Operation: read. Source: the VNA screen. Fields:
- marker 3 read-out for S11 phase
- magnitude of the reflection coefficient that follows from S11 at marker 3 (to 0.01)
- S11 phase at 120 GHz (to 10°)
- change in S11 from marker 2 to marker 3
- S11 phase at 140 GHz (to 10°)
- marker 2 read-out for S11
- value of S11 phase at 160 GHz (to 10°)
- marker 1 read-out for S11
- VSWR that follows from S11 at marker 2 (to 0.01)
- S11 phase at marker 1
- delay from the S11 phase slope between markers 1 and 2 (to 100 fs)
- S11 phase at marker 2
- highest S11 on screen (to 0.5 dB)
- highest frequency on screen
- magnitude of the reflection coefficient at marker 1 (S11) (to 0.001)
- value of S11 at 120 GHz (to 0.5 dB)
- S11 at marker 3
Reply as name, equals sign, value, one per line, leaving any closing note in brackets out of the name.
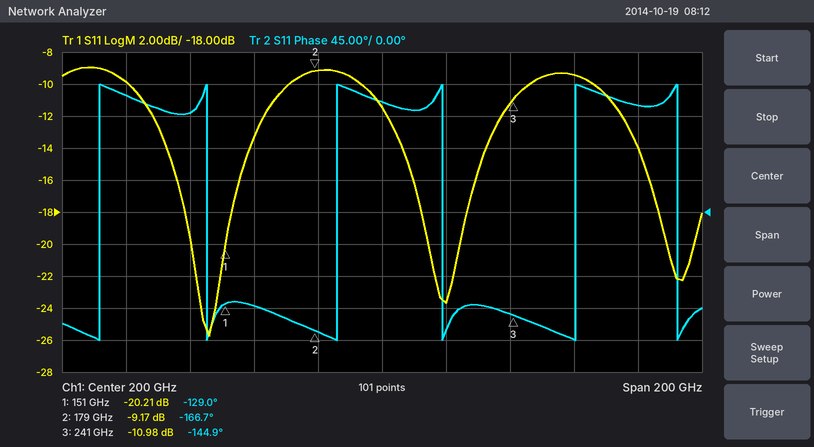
marker 3 read-out for S11 phase = -144.9°
magnitude of the reflection coefficient that follows from S11 at marker 3 = 0.28
S11 phase at 120 GHz = 160°
change in S11 from marker 2 to marker 3 = -1.81 dB
S11 phase at 140 GHz = 140°
marker 2 read-out for S11 = -9.17 dB
value of S11 phase at 160 GHz = -130°
marker 1 read-out for S11 = -20.21 dB
VSWR that follows from S11 at marker 2 = 2.07
S11 phase at marker 1 = -129.0°
delay from the S11 phase slope between markers 1 and 2 = 3.7 ps
S11 phase at marker 2 = -166.7°
highest S11 on screen = -9.0 dB
highest frequency on screen = 300 GHz
magnitude of the reflection coefficient at marker 1 (S11) = 0.098
value of S11 at 120 GHz = -10.0 dB
S11 at marker 3 = -10.98 dB
